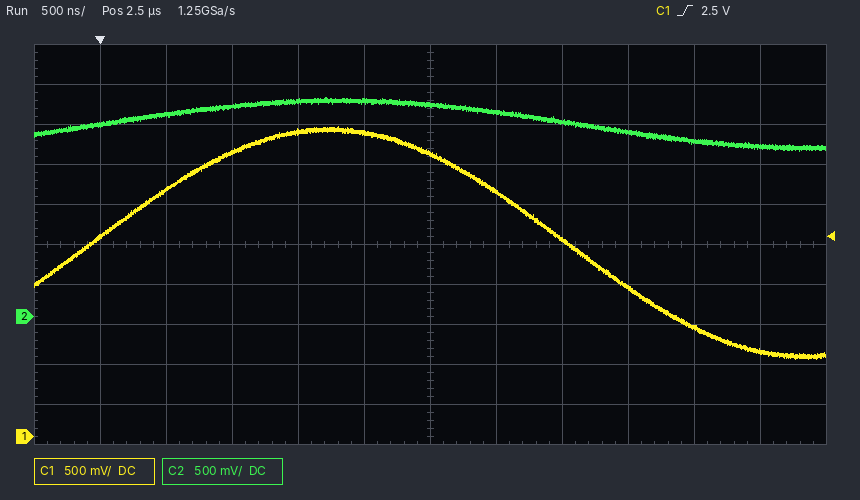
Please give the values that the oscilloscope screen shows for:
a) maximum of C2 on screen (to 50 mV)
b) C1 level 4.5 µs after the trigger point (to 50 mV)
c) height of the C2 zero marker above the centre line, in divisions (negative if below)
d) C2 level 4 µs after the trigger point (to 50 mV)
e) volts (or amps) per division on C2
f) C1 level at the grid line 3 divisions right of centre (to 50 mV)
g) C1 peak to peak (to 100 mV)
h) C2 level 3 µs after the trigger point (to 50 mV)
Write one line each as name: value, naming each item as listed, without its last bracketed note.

maximum of C2 on screen: 2.75 V
C1 level 4.5 µs after the trigger point: 1.35 V
height of the C2 zero marker above the centre line, in divisions: -1.8 div
C2 level 4 µs after the trigger point: 2.30 V
volts (or amps) per division on C2: 500 mV
C1 level at the grid line 3 divisions right of centre: 1.85 V
C1 peak to peak: 2.90 V
C2 level 3 µs after the trigger point: 2.55 V
